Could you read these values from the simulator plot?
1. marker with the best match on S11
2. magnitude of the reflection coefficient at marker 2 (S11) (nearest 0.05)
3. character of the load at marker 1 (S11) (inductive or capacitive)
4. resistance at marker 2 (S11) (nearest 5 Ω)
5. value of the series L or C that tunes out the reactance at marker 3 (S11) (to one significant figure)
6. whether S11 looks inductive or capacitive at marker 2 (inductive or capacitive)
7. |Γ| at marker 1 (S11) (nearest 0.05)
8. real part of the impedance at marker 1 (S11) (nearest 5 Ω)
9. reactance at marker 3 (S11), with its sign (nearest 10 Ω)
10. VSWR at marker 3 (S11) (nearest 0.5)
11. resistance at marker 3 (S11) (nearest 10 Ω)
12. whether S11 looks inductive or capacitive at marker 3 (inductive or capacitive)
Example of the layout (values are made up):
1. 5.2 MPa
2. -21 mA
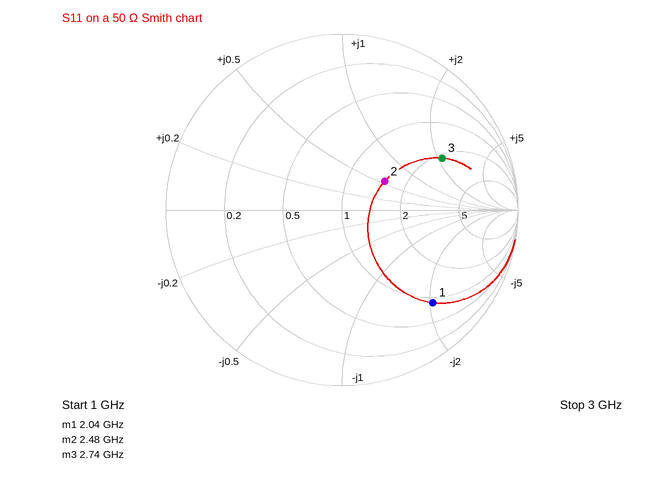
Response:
1. marker 2
2. 0.30
3. capacitive
4. 75 Ω
5. 500 fF
6. inductive
7. 0.75
8. 45 Ω
9. +110 Ω
10. 4.5
11. 110 Ω
12. inductive
